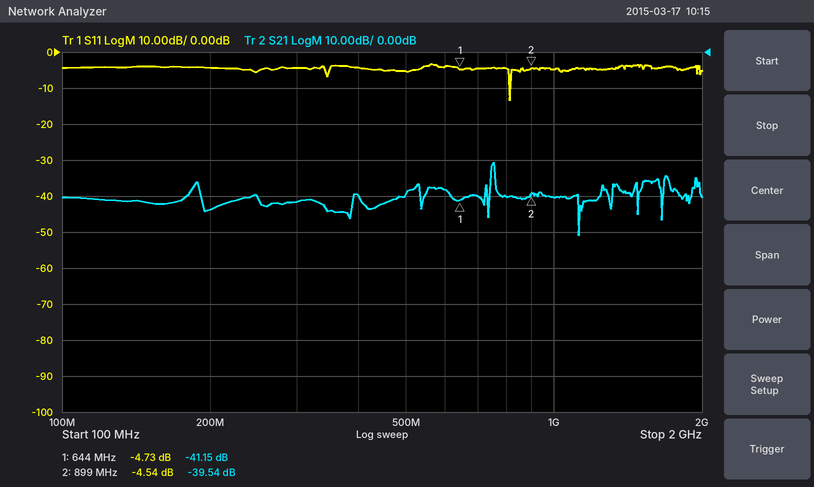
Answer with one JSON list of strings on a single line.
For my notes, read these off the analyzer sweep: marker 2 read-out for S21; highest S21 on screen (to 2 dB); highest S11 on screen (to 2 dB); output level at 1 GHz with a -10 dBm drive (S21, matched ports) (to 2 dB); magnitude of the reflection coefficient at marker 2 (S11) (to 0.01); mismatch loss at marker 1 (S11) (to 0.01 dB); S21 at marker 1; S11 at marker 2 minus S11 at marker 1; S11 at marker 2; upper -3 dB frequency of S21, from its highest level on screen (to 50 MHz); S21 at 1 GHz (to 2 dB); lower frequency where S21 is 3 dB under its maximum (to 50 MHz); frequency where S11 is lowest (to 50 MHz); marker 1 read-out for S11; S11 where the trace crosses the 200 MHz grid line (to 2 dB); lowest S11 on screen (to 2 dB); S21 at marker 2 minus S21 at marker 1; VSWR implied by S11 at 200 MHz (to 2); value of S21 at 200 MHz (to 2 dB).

["-39.54 dB", "-30 dB", "-4 dB", "-50 dBm", "0.59", "1.78 dB", "-41.15 dB", "0.19 dB", "-4.54 dB", "750 MHz", "-40 dB", "750 MHz", "800 MHz", "-4.73 dB", "-4 dB", "-14 dB", "1.61 dB", "4", "-44 dB"]
